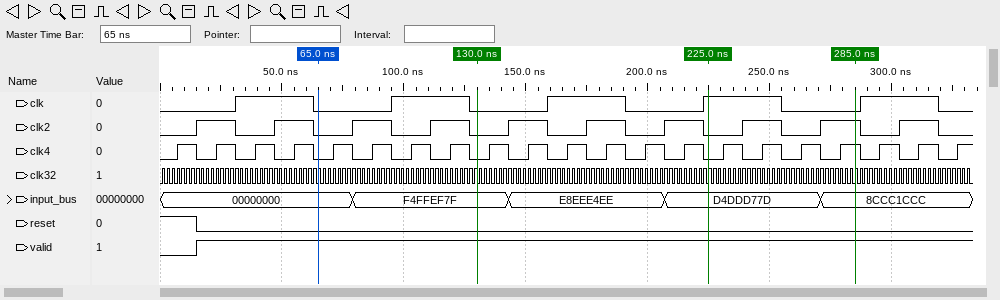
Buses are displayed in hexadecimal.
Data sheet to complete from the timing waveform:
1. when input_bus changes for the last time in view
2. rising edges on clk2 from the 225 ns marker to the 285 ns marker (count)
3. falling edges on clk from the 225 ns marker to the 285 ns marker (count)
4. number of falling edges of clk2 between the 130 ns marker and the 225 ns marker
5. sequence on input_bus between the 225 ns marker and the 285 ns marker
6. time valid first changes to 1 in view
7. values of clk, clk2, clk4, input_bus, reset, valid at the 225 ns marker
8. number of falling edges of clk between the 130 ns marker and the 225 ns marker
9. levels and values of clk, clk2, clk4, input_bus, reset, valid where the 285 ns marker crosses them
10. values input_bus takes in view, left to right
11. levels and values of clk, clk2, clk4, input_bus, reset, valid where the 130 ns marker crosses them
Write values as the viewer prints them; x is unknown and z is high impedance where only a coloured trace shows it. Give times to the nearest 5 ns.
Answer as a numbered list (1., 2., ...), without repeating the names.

1. 270 ns
2. 2
3. 1
4. 3
5. D4DDD77D, 8CCC1CCC
6. 15 ns
7. clk=1, clk2=0, clk4=0, input_bus=D4DDD77D, reset=0, valid=1
8. 1
9. clk=0, clk2=1, clk4=1, input_bus=8CCC1CCC, reset=0, valid=1
10. 00000000, F4FFEF7F, E8EEE4EE, D4DDD77D, 8CCC1CCC
11. clk=0, clk2=0, clk4=0, input_bus=F4FFEF7F, reset=0, valid=1
